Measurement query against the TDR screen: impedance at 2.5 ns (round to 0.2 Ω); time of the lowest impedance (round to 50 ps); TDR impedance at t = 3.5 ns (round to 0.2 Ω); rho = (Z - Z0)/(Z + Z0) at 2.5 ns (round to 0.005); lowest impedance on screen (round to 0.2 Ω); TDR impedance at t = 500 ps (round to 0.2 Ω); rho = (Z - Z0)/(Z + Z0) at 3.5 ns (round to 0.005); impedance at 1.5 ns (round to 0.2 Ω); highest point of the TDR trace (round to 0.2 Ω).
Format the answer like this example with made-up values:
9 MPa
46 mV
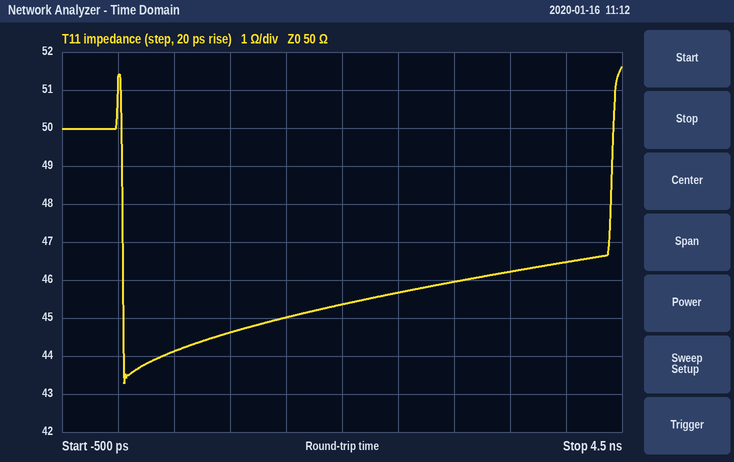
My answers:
45.6 Ω
50 ps
46.2 Ω
-0.045
43.2 Ω
44.2 Ω
-0.040
45.0 Ω
51.6 Ω
